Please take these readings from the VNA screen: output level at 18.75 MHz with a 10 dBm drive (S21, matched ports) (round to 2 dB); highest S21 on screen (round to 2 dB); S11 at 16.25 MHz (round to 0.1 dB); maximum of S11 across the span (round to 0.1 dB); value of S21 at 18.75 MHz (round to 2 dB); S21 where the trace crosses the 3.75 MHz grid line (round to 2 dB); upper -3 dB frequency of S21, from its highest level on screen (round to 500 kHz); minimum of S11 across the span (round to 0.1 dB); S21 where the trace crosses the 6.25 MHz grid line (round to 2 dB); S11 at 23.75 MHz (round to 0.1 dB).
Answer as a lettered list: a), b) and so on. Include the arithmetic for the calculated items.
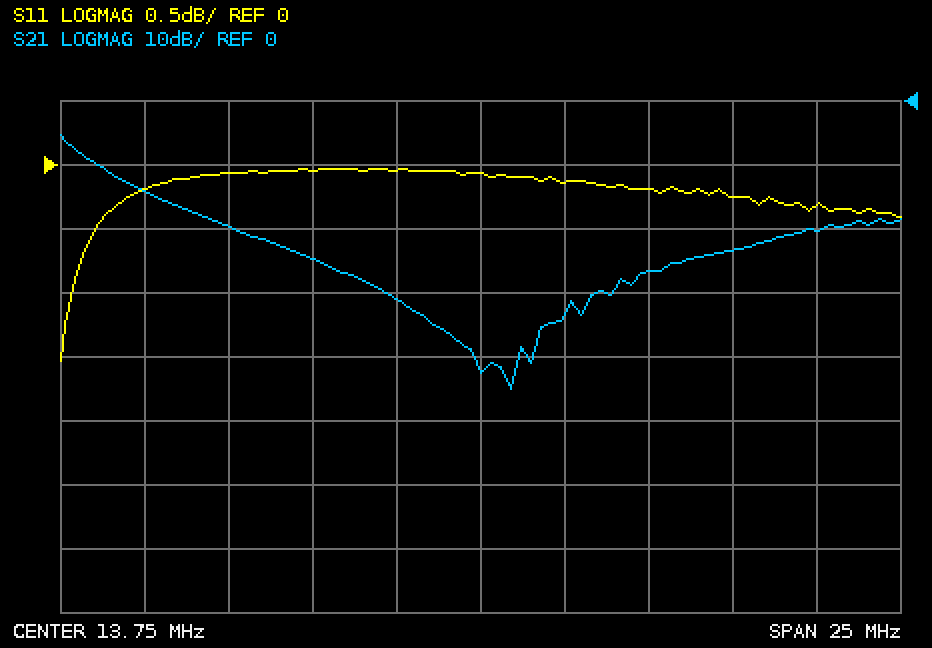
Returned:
a) 10 dBm + (-26 dB) = -16 dBm
b) -6 dB
c) -0.1 dB
d) 0.0 dB
e) -26 dB
f) -14 dB
g) 2.0 MHz
h) -1.5 dB
i) -20 dB
j) -0.3 dB
